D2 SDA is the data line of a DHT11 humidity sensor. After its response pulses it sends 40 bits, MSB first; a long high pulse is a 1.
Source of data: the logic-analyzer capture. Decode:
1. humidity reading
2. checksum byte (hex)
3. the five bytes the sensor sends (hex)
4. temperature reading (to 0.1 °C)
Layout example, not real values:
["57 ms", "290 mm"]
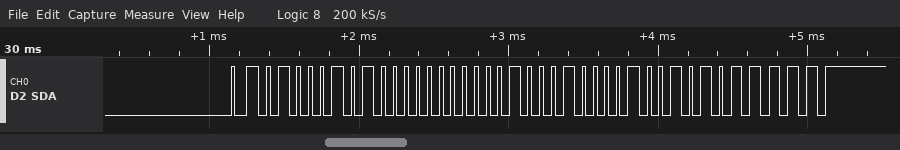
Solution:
["69 %", "0x5F", "45 00 11 09 5F", "17.9 °C"]
